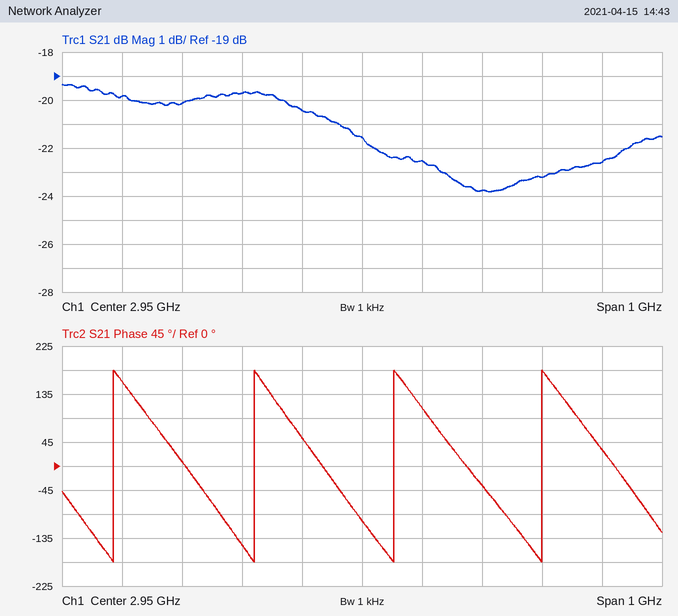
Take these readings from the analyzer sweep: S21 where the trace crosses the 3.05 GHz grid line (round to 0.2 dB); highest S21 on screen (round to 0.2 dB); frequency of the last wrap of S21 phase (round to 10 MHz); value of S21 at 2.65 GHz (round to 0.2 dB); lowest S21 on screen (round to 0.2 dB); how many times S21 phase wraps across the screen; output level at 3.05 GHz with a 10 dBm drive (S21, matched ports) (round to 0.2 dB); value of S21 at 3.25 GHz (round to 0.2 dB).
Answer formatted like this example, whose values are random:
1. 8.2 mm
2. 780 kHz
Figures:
1. -22.6 dB
2. -19.4 dB
3. 3.25 GHz
4. -20.2 dB
5. -23.8 dB
6. 4
7. -12.6 dBm
8. -23.2 dB
